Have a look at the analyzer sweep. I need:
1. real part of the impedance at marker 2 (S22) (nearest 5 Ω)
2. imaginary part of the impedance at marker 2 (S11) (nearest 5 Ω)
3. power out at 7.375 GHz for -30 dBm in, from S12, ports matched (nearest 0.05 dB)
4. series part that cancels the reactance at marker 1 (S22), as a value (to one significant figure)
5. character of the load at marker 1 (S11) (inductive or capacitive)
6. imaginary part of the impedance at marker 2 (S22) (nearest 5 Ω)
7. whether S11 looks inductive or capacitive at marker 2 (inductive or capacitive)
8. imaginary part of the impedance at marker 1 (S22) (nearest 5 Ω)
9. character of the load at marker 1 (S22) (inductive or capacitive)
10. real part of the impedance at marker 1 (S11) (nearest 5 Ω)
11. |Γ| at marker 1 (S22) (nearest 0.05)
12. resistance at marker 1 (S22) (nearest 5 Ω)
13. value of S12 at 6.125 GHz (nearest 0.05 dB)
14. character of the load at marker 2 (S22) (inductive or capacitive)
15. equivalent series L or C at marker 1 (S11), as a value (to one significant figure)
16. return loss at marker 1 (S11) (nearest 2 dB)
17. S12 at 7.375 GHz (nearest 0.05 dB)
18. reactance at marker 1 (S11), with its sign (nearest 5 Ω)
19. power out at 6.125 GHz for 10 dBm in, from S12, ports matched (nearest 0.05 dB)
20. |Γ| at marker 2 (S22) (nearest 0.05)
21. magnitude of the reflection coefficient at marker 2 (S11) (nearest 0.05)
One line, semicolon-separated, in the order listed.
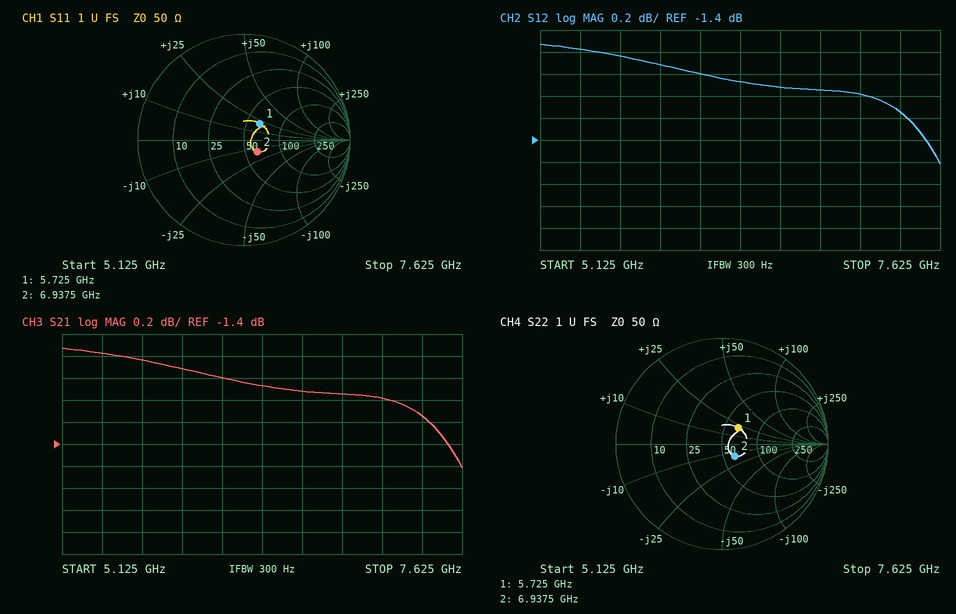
60 Ω; -15 Ω; -31.15 dBm; 1 pF; inductive; -15 Ω; capacitive; +20 Ω; inductive; 65 Ω; 0.20; 65 Ω; -0.80 dB; capacitive; 600 pH; 14 dB; -1.15 dB; +20 Ω; 9.20 dBm; 0.15; 0.15
